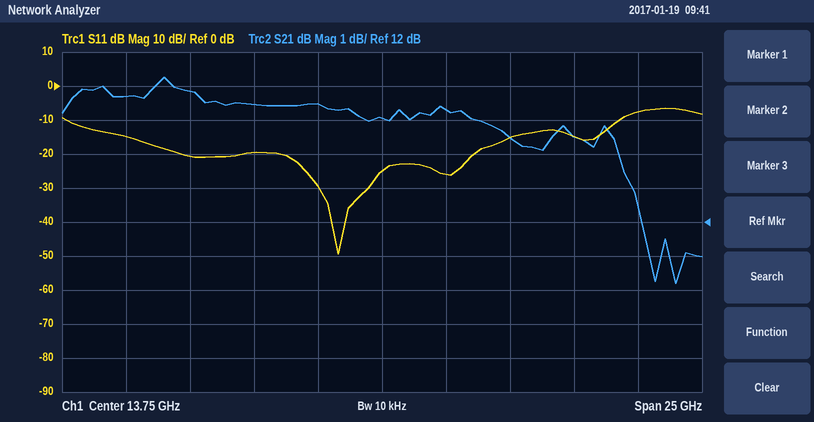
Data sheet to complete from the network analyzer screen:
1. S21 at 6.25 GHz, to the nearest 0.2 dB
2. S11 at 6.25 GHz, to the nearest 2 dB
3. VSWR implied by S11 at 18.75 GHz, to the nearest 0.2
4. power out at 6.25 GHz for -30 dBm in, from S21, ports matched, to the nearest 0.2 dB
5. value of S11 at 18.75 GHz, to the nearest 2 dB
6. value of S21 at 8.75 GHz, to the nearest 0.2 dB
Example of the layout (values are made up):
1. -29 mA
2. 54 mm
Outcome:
1. 15.8 dB
2. -20 dB
3. 1.4
4. -14.2 dBm
5. -16 dB
6. 15.4 dB
